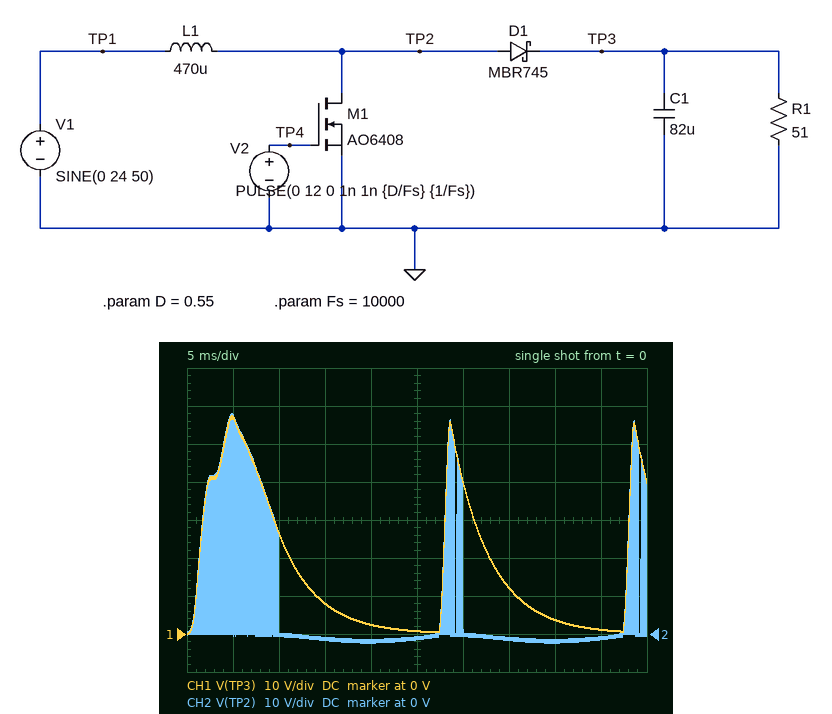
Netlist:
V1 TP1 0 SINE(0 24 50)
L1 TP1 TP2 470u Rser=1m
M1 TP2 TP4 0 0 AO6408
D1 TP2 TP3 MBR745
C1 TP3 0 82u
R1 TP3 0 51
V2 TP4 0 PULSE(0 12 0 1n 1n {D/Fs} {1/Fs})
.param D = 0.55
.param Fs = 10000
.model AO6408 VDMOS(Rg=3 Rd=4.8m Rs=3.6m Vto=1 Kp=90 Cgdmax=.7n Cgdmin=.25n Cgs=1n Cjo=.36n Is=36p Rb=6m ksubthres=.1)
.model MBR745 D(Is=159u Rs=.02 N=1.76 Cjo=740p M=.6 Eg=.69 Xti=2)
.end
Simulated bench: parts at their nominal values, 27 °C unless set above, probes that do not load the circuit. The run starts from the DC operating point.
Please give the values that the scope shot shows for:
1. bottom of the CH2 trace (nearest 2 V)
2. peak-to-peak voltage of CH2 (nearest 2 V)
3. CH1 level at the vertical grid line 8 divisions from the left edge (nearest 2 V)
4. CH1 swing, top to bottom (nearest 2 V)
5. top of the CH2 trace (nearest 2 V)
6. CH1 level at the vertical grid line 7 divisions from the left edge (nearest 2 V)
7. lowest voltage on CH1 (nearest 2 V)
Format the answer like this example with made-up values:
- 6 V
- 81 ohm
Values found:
- -2 V
- 60 V
- 4 V
- 58 V
- 58 V
- 12 V
- 0 V
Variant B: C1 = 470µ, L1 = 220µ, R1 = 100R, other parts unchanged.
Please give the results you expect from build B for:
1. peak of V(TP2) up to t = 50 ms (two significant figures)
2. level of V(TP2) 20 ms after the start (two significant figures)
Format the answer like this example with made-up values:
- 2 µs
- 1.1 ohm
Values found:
- 63 V
- -3.5 V
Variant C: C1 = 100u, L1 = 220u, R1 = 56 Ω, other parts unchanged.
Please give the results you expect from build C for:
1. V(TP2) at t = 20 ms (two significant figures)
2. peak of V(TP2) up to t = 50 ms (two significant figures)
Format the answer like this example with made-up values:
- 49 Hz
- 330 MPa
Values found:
- -3.5 V
- 75 V
